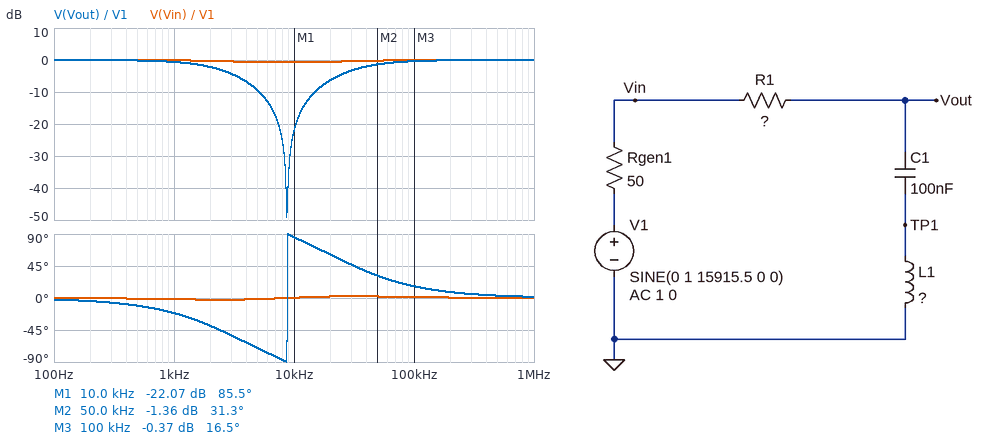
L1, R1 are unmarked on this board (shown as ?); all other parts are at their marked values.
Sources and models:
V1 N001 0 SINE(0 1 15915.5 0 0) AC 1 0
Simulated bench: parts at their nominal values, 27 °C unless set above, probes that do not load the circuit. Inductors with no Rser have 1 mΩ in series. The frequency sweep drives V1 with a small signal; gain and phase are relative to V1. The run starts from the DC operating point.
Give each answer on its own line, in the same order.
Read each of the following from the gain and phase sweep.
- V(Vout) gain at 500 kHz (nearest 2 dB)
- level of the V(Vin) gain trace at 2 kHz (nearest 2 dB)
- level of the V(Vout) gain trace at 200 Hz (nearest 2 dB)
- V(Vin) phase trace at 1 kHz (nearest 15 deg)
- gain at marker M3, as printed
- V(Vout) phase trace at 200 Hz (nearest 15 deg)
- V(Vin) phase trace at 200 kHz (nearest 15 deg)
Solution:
0 dB
0 dB
0 dB
0 deg
-0.37 dB
0 deg
0 deg
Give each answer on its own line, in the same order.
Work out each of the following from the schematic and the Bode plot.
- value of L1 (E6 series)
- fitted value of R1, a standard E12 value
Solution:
3.3 mH
560 Ω
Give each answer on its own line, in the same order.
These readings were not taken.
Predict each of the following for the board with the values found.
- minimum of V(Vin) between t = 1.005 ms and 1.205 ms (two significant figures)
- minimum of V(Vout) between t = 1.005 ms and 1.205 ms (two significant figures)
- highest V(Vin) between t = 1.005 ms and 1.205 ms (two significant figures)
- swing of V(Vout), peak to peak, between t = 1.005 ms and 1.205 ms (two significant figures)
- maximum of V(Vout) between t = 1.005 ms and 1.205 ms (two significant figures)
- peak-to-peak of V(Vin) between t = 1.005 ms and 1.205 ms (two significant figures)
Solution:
-930 mV
-350 mV
930 mV
710 mV
350 mV
1.9 V
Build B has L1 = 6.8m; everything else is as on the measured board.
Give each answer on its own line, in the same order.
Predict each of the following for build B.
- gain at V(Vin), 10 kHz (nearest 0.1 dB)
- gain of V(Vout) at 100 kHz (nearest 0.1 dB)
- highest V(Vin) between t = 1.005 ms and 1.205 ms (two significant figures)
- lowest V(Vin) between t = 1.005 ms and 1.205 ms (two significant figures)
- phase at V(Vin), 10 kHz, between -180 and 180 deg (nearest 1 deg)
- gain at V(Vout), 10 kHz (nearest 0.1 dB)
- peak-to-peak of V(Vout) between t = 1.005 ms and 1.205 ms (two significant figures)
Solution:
-0.6 dB
-0.1 dB
960 mV
-960 mV
2 deg
-7.9 dB
1.4 V
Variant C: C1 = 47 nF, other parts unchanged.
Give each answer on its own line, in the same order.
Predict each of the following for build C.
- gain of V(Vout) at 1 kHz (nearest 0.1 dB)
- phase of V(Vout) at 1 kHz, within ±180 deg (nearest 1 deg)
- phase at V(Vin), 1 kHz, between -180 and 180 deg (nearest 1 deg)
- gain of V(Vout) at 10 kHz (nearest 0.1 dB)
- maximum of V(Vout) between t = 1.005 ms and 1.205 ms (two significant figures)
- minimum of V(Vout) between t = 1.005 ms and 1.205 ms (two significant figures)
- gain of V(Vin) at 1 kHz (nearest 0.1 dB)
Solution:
-0.1 dB
-10 deg
-1 deg
-13.5 dB
190 mV
-190 mV
0 dB
